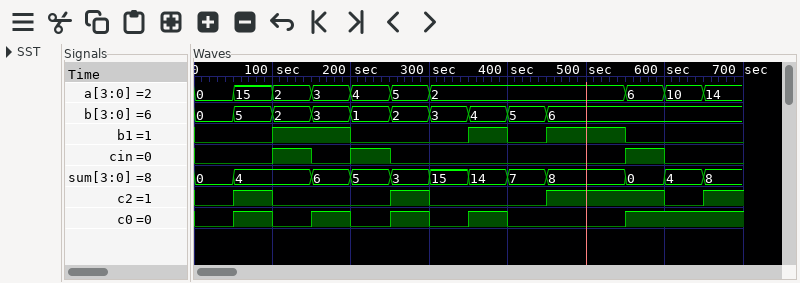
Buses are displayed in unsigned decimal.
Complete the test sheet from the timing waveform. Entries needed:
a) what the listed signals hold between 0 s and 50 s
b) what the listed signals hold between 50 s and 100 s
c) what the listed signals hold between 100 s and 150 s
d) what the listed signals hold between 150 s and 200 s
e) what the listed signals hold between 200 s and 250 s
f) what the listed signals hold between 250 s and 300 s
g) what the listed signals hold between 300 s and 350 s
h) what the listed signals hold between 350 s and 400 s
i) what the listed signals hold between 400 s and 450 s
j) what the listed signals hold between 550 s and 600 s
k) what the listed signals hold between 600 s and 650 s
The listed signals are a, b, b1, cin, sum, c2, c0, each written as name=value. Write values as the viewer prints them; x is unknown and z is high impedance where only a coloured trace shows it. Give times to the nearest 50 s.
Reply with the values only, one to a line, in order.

a=0, b=0, b1=0, cin=0, sum=0, c2=0, c0=0
a=15, b=5, b1=0, cin=0, sum=4, c2=1, c0=1
a=2, b=2, b1=1, cin=1, sum=4, c2=0, c0=0
a=3, b=3, b1=1, cin=0, sum=6, c2=0, c0=1
a=4, b=1, b1=0, cin=1, sum=5, c2=0, c0=0
a=5, b=2, b1=0, cin=0, sum=3, c2=1, c0=1
a=2, b=3, b1=0, cin=0, sum=15, c2=0, c0=0
a=2, b=4, b1=1, cin=0, sum=14, c2=0, c0=1
a=2, b=5, b1=0, cin=0, sum=7, c2=0, c0=0
a=6, b=6, b1=0, cin=1, sum=0, c2=1, c0=1
a=10, b=6, b1=0, cin=0, sum=4, c2=0, c0=1
